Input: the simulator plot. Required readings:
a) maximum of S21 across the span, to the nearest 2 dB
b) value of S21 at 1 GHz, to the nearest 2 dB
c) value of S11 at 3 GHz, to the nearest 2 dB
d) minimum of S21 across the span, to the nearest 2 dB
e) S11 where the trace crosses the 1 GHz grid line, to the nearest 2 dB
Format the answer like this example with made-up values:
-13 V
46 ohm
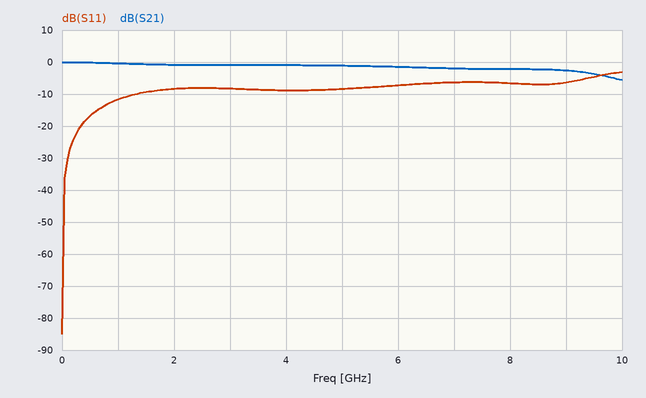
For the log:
0 dB
0 dB
-8 dB
-6 dB
-12 dB
